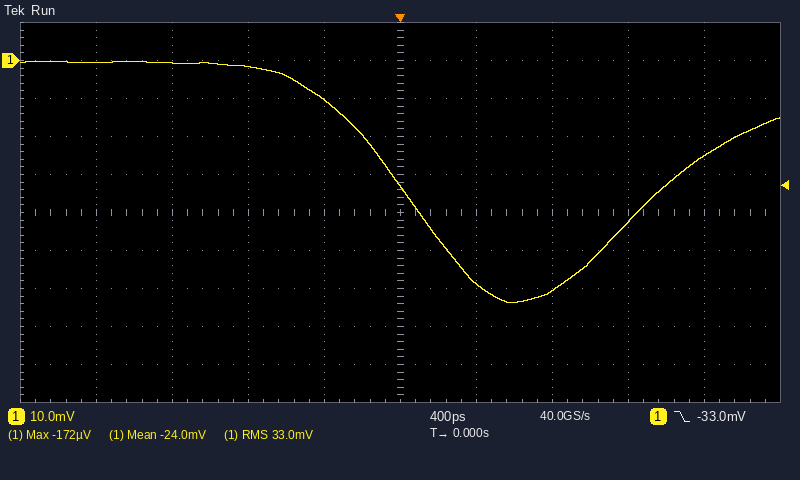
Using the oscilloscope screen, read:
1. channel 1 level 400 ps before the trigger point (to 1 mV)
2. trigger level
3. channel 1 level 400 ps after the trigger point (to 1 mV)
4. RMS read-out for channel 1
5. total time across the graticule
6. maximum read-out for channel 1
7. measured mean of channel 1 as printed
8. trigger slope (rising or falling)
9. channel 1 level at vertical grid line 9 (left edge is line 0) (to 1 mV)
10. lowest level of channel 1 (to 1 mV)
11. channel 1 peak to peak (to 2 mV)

-10 mV
-33.0 mV
-59 mV
33.0 mV
4 ns
-172 µV
-24.0 mV
falling
-25 mV
-64 mV
64 mV
